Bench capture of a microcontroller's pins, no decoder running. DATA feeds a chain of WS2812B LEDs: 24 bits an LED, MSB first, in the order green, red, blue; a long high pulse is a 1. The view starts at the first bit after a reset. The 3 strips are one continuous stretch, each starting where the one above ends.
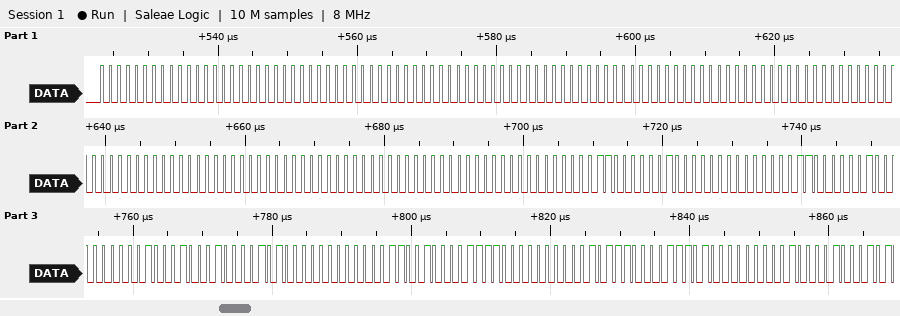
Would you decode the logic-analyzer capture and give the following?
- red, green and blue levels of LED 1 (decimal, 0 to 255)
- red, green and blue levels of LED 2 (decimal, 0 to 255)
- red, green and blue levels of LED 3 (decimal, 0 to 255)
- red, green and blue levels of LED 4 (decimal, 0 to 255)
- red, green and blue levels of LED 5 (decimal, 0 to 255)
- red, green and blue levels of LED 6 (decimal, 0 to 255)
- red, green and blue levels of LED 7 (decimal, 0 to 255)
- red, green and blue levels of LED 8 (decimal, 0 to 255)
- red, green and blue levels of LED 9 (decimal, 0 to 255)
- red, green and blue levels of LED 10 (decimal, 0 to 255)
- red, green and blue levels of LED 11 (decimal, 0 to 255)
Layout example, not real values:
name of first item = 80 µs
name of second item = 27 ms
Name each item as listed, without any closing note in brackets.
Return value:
red, green and blue levels of LED 1 = 0, 0, 0
red, green and blue levels of LED 2 = 0, 0, 0
red, green and blue levels of LED 3 = 0, 0, 0
red, green and blue levels of LED 4 = 0, 0, 0
red, green and blue levels of LED 5 = 0, 0, 0
red, green and blue levels of LED 6 = 0, 0, 0
red, green and blue levels of LED 7 = 2, 3, 0
red, green and blue levels of LED 8 = 4, 6, 1
red, green and blue levels of LED 9 = 10, 17, 0
red, green and blue levels of LED 10 = 15, 25, 0
red, green and blue levels of LED 11 = 29, 46, 0
